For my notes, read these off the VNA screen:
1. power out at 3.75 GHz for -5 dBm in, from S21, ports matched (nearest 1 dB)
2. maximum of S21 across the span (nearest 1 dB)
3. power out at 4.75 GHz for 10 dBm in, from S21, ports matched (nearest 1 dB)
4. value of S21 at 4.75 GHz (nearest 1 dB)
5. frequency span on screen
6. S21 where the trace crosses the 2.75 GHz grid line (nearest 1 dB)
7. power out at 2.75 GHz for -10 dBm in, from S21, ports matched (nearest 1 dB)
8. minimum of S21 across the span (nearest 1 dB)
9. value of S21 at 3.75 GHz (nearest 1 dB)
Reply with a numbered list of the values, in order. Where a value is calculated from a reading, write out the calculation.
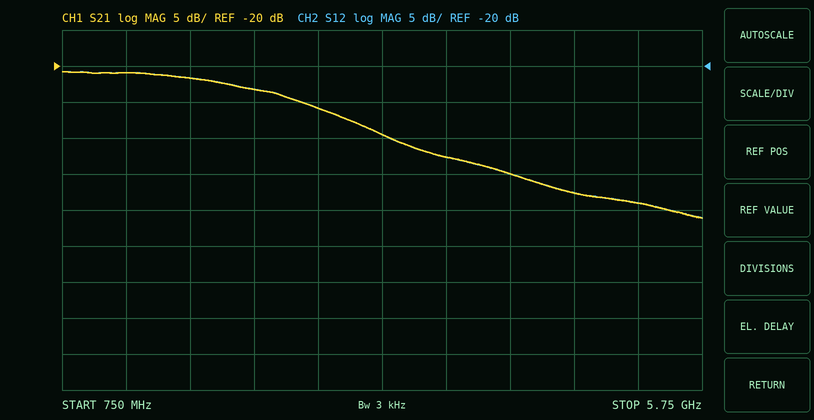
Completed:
1. -5 dBm + (-33 dB) = -38 dBm
2. -21 dB
3. 10 dBm + (-38 dB) = -28 dBm
4. -38 dB
5. 5 GHz
6. -26 dB
7. -10 dBm + (-26 dB) = -36 dBm
8. -41 dB
9. -33 dB
